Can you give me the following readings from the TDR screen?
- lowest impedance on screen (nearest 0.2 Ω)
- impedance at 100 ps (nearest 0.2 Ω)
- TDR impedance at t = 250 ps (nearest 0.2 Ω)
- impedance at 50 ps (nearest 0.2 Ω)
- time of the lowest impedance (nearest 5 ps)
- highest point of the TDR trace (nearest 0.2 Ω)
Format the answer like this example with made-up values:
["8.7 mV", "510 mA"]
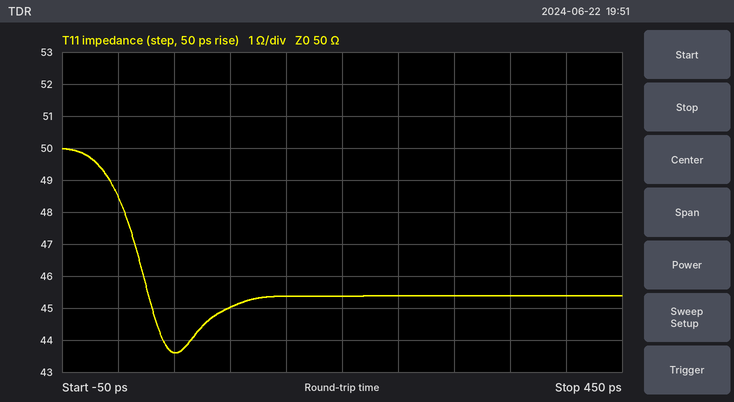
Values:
["43.6 Ω", "45.0 Ω", "45.4 Ω", "43.6 Ω", "50 ps", "50.0 Ω"]
